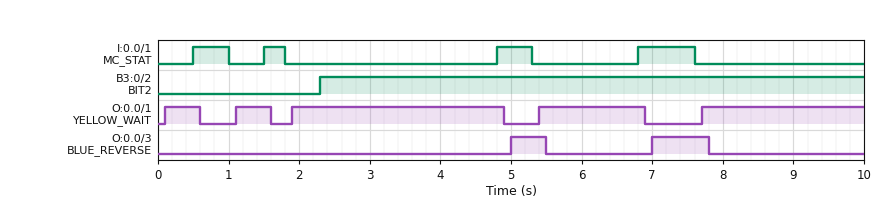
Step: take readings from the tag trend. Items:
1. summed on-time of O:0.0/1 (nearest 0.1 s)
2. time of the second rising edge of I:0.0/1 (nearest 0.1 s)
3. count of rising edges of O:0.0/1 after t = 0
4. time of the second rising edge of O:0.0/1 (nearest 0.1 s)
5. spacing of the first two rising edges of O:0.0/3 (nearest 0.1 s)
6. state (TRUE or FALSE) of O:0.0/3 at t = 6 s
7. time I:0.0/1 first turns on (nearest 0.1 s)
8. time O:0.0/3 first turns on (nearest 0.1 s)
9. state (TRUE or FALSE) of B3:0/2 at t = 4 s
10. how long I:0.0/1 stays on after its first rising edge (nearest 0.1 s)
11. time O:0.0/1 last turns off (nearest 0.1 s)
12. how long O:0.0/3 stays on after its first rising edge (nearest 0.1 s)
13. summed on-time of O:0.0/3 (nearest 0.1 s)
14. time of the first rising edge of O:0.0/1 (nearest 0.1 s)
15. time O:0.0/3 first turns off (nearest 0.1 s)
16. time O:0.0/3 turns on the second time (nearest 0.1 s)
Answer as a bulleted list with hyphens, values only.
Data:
- 7.8 s
- 1.5 s
- 5
- 1.1 s
- 2.0 s
- FALSE
- 0.5 s
- 5.0 s
- TRUE
- 0.5 s
- 6.9 s
- 0.5 s
- 1.3 s
- 0.1 s
- 5.5 s
- 7.0 s
